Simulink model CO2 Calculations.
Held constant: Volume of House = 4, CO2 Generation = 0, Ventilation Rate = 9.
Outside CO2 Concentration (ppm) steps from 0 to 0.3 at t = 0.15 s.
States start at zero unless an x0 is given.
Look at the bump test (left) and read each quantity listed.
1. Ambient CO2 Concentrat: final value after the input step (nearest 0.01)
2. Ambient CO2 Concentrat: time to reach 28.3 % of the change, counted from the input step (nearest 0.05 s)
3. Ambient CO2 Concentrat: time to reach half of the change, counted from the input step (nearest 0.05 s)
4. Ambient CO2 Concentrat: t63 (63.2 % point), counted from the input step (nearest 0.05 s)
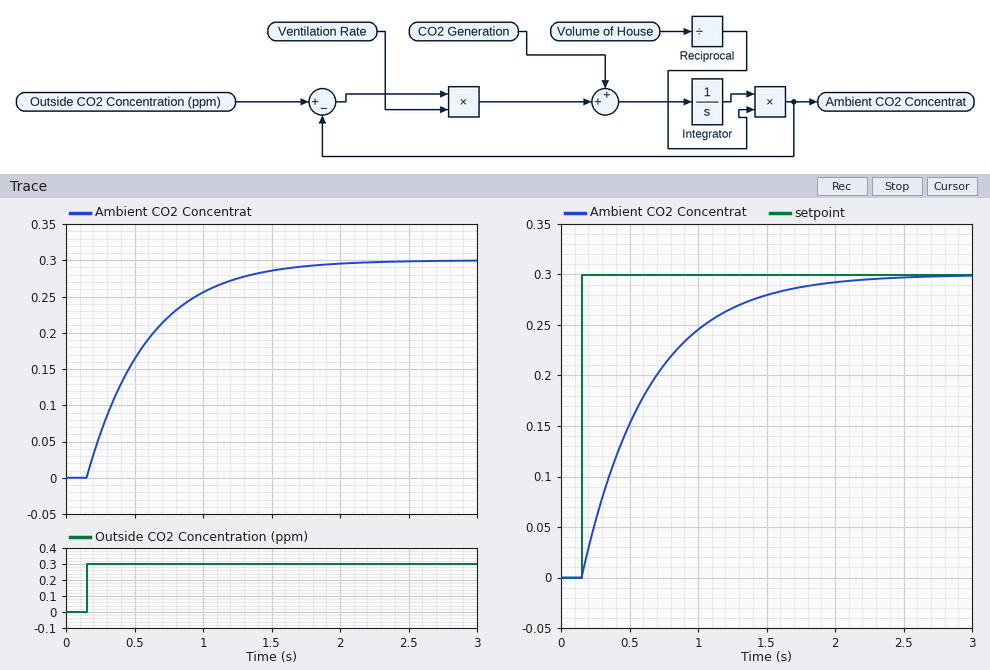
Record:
0.30
0.15 s
0.30 s
0.45 s
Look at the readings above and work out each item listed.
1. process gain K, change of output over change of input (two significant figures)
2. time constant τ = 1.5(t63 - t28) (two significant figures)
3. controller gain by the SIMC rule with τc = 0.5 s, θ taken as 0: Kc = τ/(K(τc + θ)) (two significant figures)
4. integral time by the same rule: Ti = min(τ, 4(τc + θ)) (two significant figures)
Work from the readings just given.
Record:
1.0
0.45 s
0.90
0.45 s
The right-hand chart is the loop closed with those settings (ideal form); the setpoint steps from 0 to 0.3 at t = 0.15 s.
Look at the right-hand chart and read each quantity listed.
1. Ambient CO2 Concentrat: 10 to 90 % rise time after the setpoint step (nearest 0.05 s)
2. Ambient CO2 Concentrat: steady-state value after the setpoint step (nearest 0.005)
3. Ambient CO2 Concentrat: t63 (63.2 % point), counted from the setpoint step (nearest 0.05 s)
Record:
1.10 s
0.300
0.50 s
